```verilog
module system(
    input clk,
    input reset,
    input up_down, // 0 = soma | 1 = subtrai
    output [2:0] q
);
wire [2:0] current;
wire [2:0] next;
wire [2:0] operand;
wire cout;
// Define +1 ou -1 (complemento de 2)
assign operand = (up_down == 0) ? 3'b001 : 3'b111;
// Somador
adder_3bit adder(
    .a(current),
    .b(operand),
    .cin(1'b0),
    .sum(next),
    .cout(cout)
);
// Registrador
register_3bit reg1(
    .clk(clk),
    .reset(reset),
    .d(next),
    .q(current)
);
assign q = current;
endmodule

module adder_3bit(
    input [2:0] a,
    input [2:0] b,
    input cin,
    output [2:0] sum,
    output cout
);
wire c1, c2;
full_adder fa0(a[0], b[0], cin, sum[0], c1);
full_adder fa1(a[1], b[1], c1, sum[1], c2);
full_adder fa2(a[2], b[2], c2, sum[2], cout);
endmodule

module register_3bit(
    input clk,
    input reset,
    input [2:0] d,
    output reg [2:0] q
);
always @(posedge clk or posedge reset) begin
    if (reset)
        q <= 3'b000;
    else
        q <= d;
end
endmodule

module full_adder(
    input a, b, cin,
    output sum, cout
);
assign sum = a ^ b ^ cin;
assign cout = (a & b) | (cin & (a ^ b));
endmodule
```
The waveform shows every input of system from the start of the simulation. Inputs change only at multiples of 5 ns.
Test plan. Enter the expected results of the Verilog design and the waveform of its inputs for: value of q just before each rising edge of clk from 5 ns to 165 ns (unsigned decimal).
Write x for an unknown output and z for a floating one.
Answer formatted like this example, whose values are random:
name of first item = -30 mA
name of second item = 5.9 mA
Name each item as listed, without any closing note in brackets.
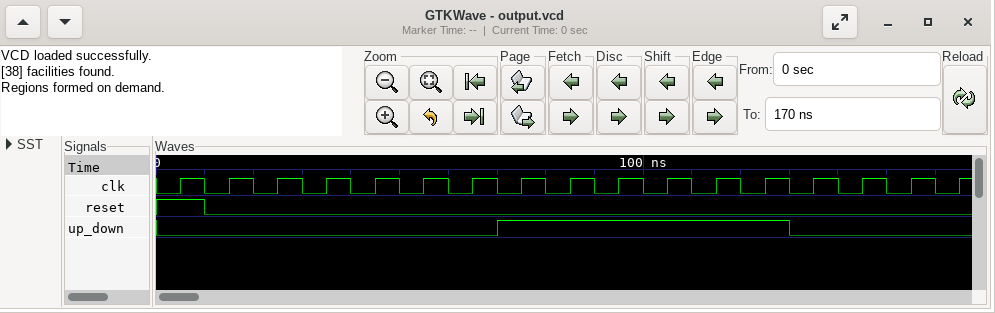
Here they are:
value of q just before each rising edge of clk from 5 ns to 165 ns = 0, 0, 1, 2, 3, 4, 5, 6, 5, 4, 3, 2, 1, 0, 1, 2, 3
